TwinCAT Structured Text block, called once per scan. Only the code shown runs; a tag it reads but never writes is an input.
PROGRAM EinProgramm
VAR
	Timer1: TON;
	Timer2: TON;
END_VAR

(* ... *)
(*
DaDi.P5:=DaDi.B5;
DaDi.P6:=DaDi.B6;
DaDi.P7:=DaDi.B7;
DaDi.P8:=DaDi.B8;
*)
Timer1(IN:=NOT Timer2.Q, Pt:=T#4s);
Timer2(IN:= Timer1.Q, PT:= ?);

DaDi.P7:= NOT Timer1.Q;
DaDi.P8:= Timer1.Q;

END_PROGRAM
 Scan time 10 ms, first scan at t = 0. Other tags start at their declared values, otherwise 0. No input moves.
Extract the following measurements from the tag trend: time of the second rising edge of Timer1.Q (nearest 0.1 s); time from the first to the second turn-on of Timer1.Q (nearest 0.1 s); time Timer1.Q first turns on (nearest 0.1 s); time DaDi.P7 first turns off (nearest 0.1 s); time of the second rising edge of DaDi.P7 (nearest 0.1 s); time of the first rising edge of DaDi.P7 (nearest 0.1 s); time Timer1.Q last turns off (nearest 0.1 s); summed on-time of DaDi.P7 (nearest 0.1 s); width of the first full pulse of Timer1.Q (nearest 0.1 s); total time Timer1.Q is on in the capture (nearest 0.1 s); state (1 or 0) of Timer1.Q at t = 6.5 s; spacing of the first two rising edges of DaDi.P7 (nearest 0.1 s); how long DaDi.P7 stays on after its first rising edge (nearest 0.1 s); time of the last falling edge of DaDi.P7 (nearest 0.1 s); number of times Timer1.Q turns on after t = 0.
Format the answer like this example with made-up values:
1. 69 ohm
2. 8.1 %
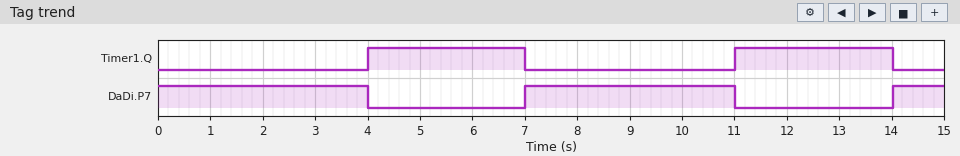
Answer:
1. 11.0 s
2. 7.0 s
3. 4.0 s
4. 4.0 s
5. 14.0 s
6. 7.0 s
7. 14.0 s
8. 9.0 s
9. 3.0 s
10. 6.0 s
11. 1
12. 7.0 s
13. 4.0 s
14. 11.0 s
15. 2
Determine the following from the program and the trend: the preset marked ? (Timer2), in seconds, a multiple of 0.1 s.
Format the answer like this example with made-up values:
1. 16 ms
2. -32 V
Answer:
1. 3.0 s
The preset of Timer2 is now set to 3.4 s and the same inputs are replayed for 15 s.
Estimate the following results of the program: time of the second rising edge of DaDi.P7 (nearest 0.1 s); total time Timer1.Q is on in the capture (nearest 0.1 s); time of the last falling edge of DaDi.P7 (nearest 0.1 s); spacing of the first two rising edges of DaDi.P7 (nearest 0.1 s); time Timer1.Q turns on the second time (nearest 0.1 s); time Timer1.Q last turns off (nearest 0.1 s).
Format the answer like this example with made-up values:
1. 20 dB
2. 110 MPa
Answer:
1. 14.8 s
2. 6.8 s
3. 11.4 s
4. 7.4 s
5. 11.4 s
6. 14.8 s
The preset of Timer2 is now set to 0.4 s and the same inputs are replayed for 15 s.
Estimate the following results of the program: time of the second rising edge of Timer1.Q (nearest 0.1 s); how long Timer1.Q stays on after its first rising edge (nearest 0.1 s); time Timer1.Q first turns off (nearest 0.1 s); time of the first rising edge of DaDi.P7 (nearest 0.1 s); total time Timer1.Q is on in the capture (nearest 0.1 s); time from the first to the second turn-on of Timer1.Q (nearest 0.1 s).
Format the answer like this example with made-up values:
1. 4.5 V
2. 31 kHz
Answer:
1. 8.4 s
2. 0.4 s
3. 4.4 s
4. 4.4 s
5. 1.2 s
6. 4.4 s
